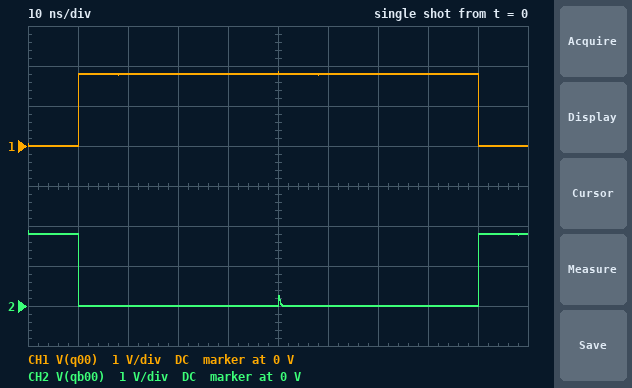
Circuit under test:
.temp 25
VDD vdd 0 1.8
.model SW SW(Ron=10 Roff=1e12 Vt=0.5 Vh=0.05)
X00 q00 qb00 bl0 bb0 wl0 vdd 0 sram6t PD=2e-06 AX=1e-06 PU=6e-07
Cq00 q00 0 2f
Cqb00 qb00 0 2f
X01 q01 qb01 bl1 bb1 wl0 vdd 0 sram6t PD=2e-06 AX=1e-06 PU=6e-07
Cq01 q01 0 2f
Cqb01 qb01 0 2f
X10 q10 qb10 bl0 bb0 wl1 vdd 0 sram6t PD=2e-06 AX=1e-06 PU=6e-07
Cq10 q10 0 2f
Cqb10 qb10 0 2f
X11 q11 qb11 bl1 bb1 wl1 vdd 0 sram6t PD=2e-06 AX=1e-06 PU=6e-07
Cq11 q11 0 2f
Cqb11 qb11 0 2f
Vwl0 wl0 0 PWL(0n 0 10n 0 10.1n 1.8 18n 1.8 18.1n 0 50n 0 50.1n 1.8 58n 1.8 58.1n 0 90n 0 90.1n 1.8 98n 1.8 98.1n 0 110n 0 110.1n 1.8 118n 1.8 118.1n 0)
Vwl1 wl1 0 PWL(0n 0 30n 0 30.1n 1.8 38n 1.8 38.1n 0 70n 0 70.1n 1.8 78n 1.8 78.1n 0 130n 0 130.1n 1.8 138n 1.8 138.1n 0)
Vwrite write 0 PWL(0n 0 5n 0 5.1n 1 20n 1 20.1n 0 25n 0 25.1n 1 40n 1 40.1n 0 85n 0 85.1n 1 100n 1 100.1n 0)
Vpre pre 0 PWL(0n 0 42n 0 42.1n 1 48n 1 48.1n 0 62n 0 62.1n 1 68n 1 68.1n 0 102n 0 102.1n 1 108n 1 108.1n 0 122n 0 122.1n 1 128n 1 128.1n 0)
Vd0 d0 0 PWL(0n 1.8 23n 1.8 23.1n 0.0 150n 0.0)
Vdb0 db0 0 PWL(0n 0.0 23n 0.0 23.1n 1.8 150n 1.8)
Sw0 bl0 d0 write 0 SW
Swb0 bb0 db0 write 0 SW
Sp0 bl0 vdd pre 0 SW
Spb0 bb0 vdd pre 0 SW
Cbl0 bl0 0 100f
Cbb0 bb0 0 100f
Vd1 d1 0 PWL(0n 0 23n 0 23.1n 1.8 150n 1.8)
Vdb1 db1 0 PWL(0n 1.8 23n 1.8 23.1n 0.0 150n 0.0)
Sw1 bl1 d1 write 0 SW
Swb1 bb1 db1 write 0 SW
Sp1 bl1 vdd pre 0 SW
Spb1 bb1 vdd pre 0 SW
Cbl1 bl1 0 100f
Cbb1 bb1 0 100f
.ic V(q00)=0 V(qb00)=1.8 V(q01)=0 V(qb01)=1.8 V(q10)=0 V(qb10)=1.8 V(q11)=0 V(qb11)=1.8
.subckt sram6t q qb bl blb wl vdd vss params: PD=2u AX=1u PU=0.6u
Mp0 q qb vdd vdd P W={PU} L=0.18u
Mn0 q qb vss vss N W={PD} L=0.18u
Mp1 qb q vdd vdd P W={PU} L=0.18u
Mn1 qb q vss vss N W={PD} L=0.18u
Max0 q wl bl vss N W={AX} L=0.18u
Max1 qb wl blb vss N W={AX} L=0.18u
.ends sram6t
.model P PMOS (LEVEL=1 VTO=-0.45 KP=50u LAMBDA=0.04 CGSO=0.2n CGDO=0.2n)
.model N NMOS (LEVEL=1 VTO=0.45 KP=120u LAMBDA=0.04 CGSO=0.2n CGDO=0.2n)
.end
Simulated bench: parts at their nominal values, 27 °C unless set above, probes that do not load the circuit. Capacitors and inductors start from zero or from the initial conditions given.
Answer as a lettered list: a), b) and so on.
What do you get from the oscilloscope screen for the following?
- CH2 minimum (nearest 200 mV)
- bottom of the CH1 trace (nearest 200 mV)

a) 0 V
b) 0 V
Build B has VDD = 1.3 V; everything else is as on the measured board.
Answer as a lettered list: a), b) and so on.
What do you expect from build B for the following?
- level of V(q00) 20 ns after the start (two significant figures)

a) 1.3 V
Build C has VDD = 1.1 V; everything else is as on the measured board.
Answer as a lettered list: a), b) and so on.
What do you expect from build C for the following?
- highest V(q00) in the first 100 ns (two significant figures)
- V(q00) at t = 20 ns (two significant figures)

a) 1.2 V
b) 1.1 V
